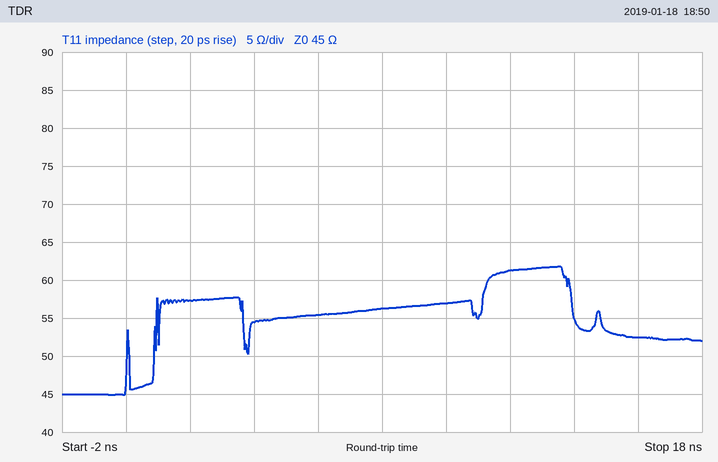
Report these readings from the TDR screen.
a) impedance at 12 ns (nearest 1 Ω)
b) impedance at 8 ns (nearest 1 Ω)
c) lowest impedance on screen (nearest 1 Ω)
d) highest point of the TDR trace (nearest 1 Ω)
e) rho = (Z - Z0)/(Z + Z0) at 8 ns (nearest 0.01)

61 Ω
56 Ω
45 Ω
62 Ω
+0.11
